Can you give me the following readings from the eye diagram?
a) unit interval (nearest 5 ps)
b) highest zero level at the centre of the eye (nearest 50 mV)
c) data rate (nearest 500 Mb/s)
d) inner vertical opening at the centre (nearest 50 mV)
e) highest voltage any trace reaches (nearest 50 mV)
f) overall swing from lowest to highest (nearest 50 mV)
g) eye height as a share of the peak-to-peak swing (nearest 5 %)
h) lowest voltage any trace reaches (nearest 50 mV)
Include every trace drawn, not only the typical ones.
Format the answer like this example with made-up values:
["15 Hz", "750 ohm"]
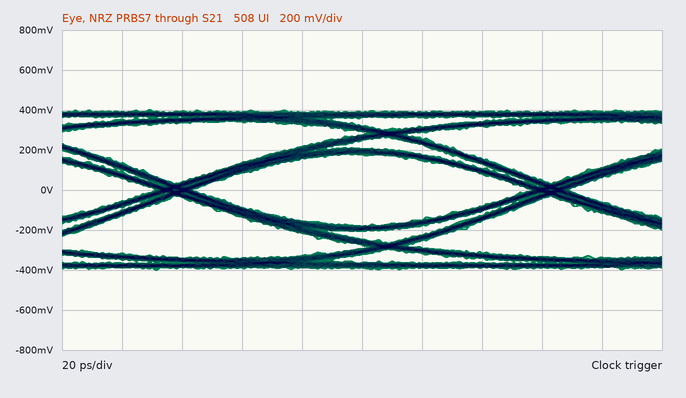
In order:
["125 ps", "-200 mV", "8.0 Gb/s", "350 mV", "400 mV", "800 mV", "45 %", "-400 mV"]
